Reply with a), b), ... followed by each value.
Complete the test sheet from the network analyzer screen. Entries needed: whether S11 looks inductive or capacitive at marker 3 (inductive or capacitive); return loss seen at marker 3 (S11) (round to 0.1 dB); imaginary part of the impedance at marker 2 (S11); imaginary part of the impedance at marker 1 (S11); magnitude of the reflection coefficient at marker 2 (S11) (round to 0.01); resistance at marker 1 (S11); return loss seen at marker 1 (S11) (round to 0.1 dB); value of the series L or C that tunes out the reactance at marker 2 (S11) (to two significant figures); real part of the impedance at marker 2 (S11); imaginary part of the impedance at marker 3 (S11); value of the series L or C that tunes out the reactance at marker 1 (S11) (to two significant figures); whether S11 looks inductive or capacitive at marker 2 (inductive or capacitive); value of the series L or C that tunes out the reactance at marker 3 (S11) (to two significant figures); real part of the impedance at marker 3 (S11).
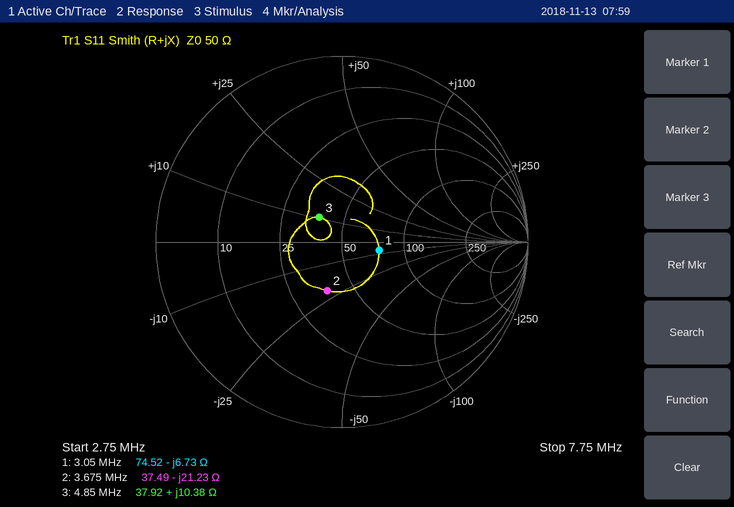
a) inductive
b) 14.9 dB
c) -21.23 Ω
d) -6.73 Ω
e) 0.27
f) 74.52 Ω
g) 13.8 dB
h) 920 nH
i) 37.49 Ω
j) +10.38 Ω
k) 350 nH
l) capacitive
m) 3.2 nF
n) 37.92 Ω
